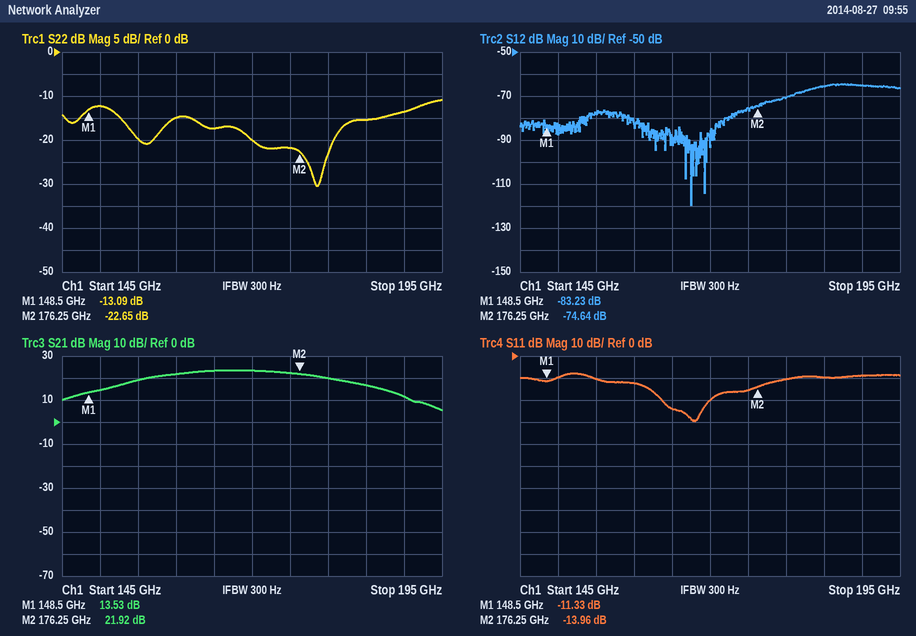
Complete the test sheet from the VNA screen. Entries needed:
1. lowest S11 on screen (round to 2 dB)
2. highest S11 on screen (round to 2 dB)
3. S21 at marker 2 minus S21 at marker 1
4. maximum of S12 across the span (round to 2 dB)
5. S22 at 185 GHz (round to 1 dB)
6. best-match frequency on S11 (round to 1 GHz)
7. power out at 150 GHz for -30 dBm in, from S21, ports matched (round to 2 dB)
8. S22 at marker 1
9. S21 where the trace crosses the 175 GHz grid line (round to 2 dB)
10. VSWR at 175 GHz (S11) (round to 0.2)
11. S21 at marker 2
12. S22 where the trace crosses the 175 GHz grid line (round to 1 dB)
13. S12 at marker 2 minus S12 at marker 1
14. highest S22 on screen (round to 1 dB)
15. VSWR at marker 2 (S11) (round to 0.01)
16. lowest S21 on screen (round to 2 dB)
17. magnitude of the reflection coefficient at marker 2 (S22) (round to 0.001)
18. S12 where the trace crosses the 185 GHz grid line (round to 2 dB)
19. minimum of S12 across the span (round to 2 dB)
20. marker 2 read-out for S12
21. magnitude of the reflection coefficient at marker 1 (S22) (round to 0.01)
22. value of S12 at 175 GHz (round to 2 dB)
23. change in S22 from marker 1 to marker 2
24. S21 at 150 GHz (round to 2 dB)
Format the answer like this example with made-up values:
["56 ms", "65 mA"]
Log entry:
["-30 dB", "-8 dB", "8.39 dB", "-64 dB", "-15 dB", "168 GHz", "-16 dBm", "-13.09 dB", "22 dB", "1.4", "21.92 dB", "-22 dB", "8.59 dB", "-11 dB", "1.50", "6 dB", "0.074", "-66 dB", "-120 dB", "-74.64 dB", "0.22", "-76 dB", "-9.56 dB", "14 dB"]
